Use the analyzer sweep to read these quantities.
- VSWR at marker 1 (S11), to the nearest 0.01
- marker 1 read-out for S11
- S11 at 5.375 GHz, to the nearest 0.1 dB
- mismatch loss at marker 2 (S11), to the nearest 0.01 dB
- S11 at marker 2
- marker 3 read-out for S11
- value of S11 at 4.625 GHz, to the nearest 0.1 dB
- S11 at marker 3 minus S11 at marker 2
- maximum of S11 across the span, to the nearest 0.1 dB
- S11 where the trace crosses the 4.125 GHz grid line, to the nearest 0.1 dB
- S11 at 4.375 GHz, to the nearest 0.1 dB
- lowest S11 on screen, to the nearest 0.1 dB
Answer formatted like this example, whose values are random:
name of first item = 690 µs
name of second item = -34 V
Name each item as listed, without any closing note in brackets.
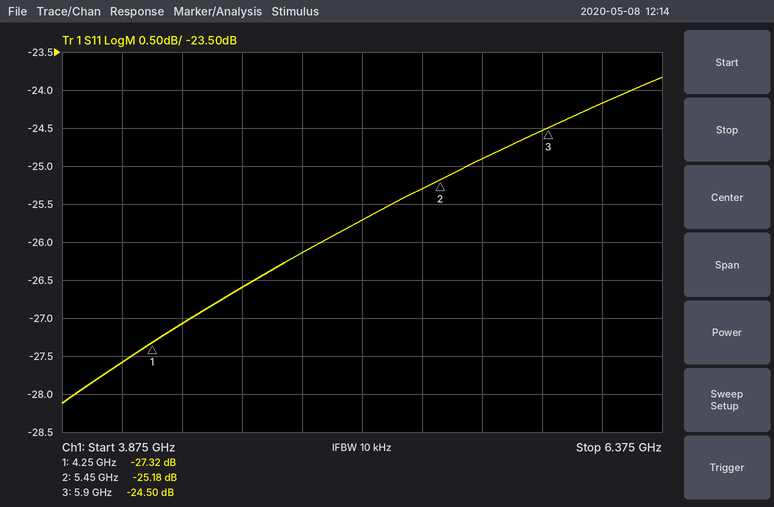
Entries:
VSWR at marker 1 (S11), to the nearest 0.01 = 1.09
marker 1 read-out for S11 = -27.32 dB
S11 at 5.375 GHz, to the nearest 0.1 dB = -25.3 dB
mismatch loss at marker 2 (S11), to the nearest 0.01 dB = 0.01 dB
S11 at marker 2 = -25.18 dB
marker 3 read-out for S11 = -24.50 dB
value of S11 at 4.625 GHz, to the nearest 0.1 dB = -26.6 dB
S11 at marker 3 minus S11 at marker 2 = 0.68 dB
maximum of S11 across the span, to the nearest 0.1 dB = -23.8 dB
S11 where the trace crosses the 4.125 GHz grid line, to the nearest 0.1 dB = -27.6 dB
S11 at 4.375 GHz, to the nearest 0.1 dB = -27.1 dB
lowest S11 on screen, to the nearest 0.1 dB = -28.1 dB
